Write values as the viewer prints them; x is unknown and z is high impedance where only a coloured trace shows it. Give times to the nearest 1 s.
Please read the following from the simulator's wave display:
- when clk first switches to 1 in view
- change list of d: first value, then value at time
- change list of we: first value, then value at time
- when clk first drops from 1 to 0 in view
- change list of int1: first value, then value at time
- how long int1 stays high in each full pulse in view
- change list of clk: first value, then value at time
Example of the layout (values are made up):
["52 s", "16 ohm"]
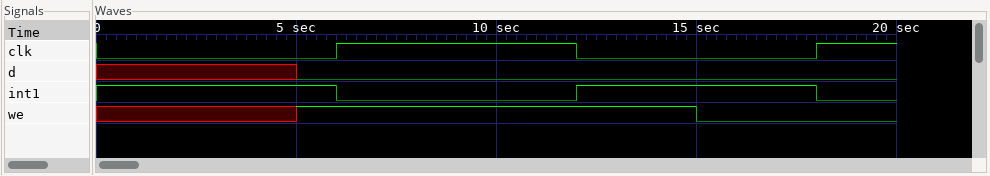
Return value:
["6 s", "x, 0 at 5 s", "x, 1 at 5 s, 0 at 15 s", "12 s", "1, 0 at 6 s, 1 at 12 s, 0 at 18 s", "6 s", "0, 1 at 6 s, 0 at 12 s, 1 at 18 s"]
